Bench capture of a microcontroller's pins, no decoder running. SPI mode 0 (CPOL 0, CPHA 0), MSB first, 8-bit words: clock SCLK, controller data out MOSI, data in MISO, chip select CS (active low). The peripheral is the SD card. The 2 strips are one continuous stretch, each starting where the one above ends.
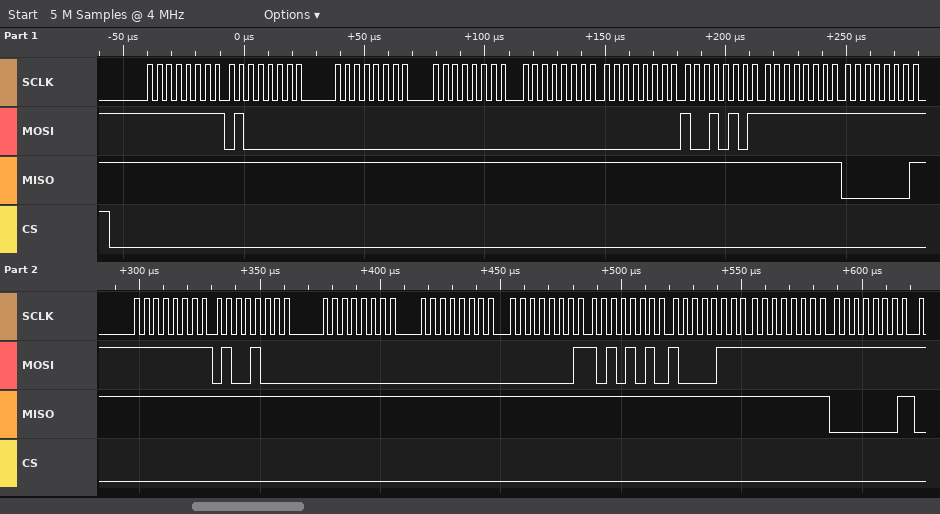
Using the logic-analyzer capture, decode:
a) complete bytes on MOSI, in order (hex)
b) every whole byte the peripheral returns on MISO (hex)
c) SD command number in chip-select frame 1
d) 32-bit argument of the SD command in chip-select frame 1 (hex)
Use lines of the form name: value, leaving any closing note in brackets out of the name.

complete bytes on MOSI, in order: 0xFF 0x40 0x00 0x00 0x00 0x00 0x95 0xFF 0xFF 0xFF 0x48 0x00 0x00 0x01 0xAA 0x87 0xFF 0xFF
every whole byte the peripheral returns on MISO: 0xFF 0xFF 0xFF 0xFF 0xFF 0xFF 0xFF 0xFF 0x01 0xFF 0xFF 0xFF 0xFF 0xFF 0xFF 0xFF 0xFF 0x01
SD command number in chip-select frame 1: CMD0
32-bit argument of the SD command in chip-select frame 1: 0x00000000
